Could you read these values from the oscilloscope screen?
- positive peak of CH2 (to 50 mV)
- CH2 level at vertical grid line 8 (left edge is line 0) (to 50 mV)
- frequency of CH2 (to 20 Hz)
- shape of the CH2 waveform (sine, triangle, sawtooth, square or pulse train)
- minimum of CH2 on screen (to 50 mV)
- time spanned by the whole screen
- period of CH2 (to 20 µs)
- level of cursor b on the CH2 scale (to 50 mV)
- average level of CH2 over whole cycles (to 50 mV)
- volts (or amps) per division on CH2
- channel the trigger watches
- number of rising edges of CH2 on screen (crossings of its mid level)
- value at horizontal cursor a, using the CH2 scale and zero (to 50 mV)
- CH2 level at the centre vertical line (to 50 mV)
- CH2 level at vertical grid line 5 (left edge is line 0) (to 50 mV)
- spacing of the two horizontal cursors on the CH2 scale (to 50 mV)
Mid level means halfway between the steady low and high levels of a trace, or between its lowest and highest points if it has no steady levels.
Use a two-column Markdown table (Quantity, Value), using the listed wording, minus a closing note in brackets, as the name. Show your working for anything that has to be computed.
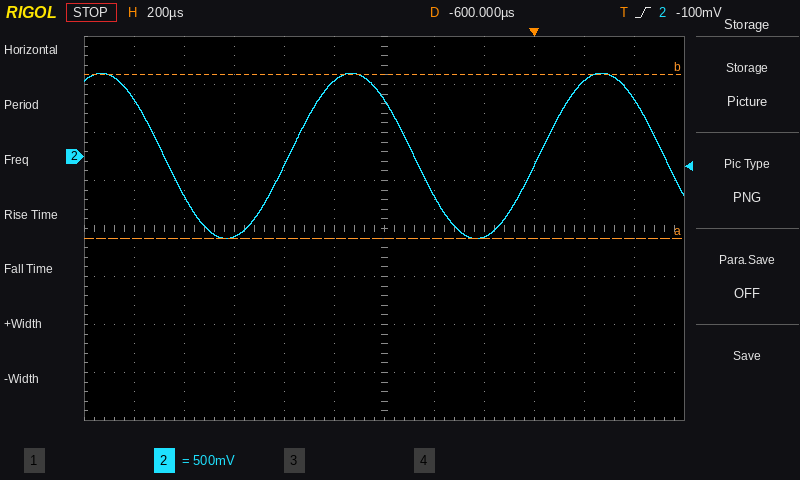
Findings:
| Quantity | Value |
|---|---|
| positive peak of CH2 | 850 mV |
| CH2 level at vertical grid line 8 (left edge is line 0) | -850 mV |
| frequency of CH2 | 1 / 1.00 ms ≈ 1.00 kHz |
| shape of the CH2 waveform | sine |
| minimum of CH2 on screen | -850 mV |
| time spanned by the whole screen | 2.4 ms |
| period of CH2 | 1.00 ms |
| level of cursor b on the CH2 scale | 850 mV |
| average level of CH2 over whole cycles | (850 mV + (-850 mV)) / 2 ≈ 0 mV |
| volts (or amps) per division on CH2 | 500 mV |
| channel the trigger watches | CH2 |
| number of rising edges of CH2 on screen | 2 |
| value at horizontal cursor a, using the CH2 scale and zero | -850 mV |
| CH2 level at the centre vertical line | 600 mV |
| CH2 level at vertical grid line 5 (left edge is line 0) | 800 mV |
| spacing of the two horizontal cursors on the CH2 scale | 1.70 V |
